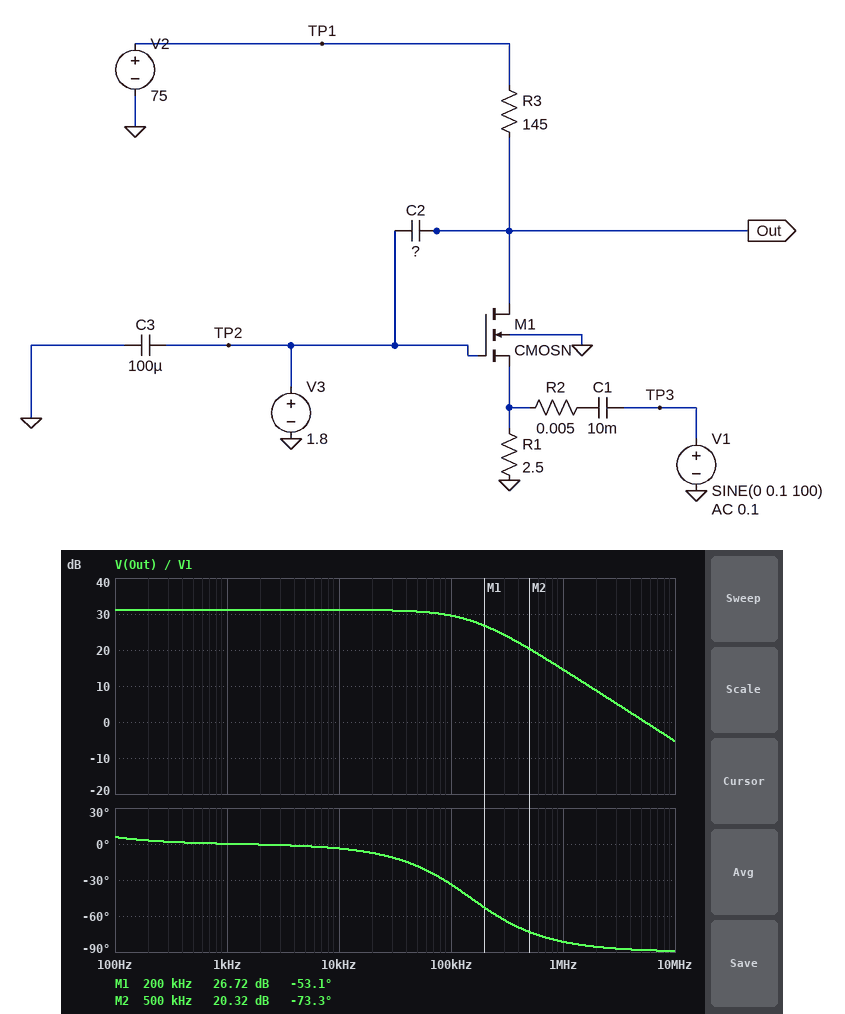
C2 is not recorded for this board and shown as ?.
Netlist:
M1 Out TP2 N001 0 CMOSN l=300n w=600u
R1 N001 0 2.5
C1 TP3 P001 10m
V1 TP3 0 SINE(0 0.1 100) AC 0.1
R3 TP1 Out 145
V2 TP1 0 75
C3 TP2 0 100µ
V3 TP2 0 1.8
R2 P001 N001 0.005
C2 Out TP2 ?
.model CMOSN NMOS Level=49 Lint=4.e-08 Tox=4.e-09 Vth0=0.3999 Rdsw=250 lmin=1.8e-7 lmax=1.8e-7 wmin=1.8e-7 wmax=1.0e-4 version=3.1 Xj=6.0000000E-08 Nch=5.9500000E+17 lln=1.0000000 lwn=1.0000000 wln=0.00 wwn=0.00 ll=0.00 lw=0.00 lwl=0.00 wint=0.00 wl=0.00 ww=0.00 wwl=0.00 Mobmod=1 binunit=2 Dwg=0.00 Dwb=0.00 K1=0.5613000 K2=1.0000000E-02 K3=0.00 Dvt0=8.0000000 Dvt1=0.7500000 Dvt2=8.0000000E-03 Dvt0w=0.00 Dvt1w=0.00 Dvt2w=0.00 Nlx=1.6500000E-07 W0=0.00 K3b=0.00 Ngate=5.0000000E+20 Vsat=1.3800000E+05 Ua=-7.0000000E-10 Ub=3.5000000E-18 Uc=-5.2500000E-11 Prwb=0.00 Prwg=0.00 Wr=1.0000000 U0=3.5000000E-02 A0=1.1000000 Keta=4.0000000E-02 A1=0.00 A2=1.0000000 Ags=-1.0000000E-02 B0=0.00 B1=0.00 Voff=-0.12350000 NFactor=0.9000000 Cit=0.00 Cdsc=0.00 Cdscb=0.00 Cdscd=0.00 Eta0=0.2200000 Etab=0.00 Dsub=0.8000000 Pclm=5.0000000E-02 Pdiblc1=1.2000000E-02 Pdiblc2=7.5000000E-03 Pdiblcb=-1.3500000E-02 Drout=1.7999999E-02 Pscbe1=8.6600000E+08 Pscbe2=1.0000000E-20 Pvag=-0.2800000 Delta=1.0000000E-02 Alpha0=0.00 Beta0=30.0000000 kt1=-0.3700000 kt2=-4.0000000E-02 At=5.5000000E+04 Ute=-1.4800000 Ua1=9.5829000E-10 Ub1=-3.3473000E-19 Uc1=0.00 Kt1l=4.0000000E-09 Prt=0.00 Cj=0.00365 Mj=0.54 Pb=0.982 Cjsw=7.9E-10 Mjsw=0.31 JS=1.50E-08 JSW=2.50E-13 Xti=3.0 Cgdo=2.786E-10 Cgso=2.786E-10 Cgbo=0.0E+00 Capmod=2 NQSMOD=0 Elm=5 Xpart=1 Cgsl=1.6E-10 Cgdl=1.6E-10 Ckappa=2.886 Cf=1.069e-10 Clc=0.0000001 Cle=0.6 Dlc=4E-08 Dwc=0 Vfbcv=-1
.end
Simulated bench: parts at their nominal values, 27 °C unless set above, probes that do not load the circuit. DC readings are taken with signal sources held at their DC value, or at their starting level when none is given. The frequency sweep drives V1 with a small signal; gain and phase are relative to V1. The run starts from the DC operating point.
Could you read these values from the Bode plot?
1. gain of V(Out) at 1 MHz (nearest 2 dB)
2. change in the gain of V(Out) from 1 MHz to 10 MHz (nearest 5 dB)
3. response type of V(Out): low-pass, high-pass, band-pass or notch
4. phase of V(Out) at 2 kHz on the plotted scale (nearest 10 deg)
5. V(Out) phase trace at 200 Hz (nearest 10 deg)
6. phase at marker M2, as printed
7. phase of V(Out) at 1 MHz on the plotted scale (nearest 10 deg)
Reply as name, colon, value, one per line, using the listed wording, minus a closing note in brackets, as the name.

gain of V(Out) at 1 MHz: 14 dB
change in the gain of V(Out) from 1 MHz to 10 MHz: -20 dB
response type of V(Out): low-pass, high-pass, band-pass or notch: low-pass
phase of V(Out) at 2 kHz on the plotted scale: 0 deg
V(Out) phase trace at 200 Hz: 0 deg
phase at marker M2, as printed: -73.3 deg
phase of V(Out) at 1 MHz on the plotted scale: -80 deg
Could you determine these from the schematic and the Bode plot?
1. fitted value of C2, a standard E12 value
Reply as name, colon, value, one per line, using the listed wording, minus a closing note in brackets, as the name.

fitted value of C2, a standard E12 value: 18 nF
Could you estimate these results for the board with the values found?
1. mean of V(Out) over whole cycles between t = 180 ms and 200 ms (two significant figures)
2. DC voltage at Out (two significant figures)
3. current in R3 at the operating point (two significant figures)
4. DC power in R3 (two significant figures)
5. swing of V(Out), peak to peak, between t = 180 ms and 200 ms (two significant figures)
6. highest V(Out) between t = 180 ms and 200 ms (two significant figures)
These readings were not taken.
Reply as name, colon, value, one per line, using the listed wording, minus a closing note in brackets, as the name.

mean of V(Out) over whole cycles between t = 180 ms and 200 ms: 34 V
DC voltage at Out: 34 V
current in R3 at the operating point: 280 mA
DC power in R3: 12 W
swing of V(Out), peak to peak, between t = 180 ms and 200 ms: 7.2 V
highest V(Out) between t = 180 ms and 200 ms: 38 V
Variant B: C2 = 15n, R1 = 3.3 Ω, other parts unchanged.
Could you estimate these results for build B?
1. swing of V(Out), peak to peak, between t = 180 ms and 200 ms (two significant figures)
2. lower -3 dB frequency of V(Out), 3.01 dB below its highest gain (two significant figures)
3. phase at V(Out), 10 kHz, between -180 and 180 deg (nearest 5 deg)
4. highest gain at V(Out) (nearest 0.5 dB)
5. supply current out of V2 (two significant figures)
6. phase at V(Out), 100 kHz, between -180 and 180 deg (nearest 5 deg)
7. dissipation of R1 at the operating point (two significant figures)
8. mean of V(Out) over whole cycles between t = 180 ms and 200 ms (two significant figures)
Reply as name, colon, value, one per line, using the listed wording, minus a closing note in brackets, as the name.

swing of V(Out), peak to peak, between t = 180 ms and 200 ms: 8.8 V
lower -3 dB frequency of V(Out), 3.01 dB below its highest gain: 9.6 Hz
phase at V(Out), 10 kHz, between -180 and 180 deg: -5 deg
highest gain at V(Out): 33.0 dB
supply current out of V2: 250 mA
phase at V(Out), 100 kHz, between -180 and 180 deg: -30 deg
dissipation of R1 at the operating point: 210 mW
mean of V(Out) over whole cycles between t = 180 ms and 200 ms: 39 V
